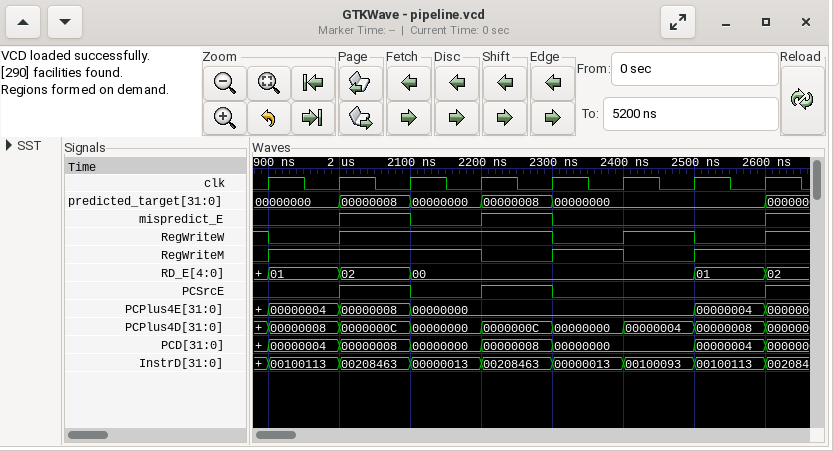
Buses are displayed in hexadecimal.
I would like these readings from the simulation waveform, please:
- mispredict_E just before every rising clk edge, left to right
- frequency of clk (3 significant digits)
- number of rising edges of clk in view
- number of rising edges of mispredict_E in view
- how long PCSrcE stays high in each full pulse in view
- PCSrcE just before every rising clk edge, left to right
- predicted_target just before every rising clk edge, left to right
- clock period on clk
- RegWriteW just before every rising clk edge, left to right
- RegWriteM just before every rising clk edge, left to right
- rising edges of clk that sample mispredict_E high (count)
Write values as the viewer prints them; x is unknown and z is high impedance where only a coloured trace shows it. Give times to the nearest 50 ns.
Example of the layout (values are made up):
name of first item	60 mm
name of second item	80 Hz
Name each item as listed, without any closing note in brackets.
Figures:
mispredict_E just before every rising clk edge, left to right	0 0 1 0 1 0 0 0
frequency of clk	10.0 MHz
number of rising edges of clk in view	8
number of rising edges of mispredict_E in view	3
how long PCSrcE stays high in each full pulse in view	100 ns, 100 ns
PCSrcE just before every rising clk edge, left to right	0 0 1 0 1 0 0 0
predicted_target just before every rising clk edge, left to right	00000000, 00000000, 00000008, 00000000, 00000008, 00000000, 00000000, 00000000
clock period on clk	100 ns
RegWriteW just before every rising clk edge, left to right	1 0 1 1 1 0 1 0
RegWriteM just before every rising clk edge, left to right	0 1 1 1 0 1 0 1
rising edges of clk that sample mispredict_E high	2
